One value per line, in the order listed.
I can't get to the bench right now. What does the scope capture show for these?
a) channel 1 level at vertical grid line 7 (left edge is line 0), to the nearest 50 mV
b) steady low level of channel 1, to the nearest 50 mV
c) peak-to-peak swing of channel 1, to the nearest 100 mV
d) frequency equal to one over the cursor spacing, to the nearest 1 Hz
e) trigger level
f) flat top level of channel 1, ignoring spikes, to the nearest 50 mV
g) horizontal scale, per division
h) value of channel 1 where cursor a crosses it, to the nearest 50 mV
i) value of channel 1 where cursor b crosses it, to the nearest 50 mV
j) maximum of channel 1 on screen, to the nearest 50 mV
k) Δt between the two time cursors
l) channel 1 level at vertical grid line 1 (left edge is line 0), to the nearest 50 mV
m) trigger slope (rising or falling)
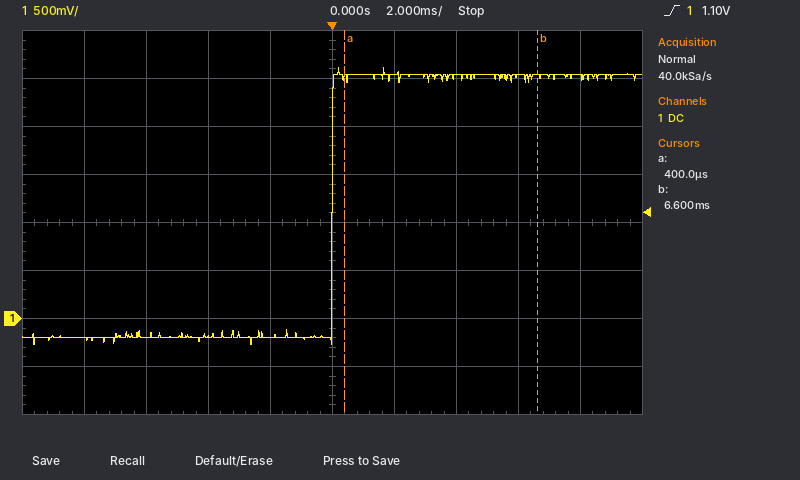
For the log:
2.50 V
-200 mV
2.90 V
161 Hz
1.10 V
2.55 V
2 ms
2.50 V
2.50 V
2.60 V
6.2 ms
-200 mV
rising
